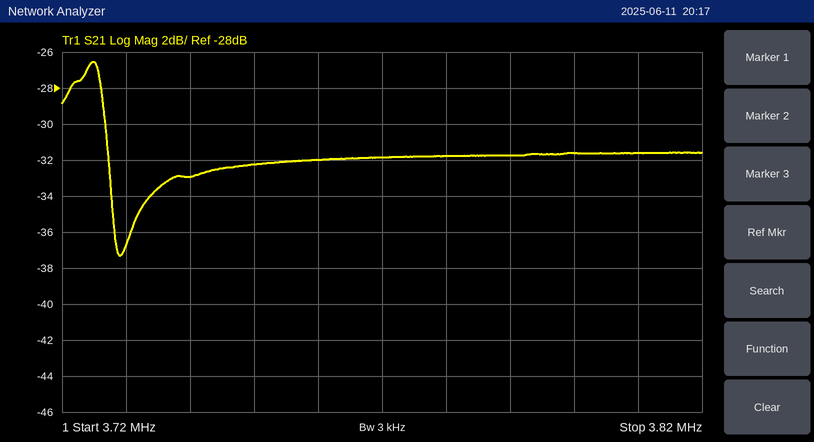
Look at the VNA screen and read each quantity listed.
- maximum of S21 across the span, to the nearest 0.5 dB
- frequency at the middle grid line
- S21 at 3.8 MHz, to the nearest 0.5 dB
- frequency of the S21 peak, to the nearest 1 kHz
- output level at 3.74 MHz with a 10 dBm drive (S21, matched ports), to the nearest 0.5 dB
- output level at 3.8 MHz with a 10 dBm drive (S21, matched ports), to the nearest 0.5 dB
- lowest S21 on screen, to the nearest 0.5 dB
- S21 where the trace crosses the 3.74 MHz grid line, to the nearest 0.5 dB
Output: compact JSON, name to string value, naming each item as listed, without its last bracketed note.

{"maximum of S21 across the span, to the nearest 0.5 dB": "-26.5 dB", "frequency at the middle grid line": "3.77 MHz", "S21 at 3.8 MHz, to the nearest 0.5 dB": "-31.5 dB", "frequency of the S21 peak, to the nearest 1 kHz": "3.725 MHz", "output level at 3.74 MHz with a 10 dBm drive (S21, matched ports), to the nearest 0.5 dB": "-23.0 dBm", "output level at 3.8 MHz with a 10 dBm drive (S21, matched ports), to the nearest 0.5 dB": "-21.5 dBm", "lowest S21 on screen, to the nearest 0.5 dB": "-37.5 dB", "S21 where the trace crosses the 3.74 MHz grid line, to the nearest 0.5 dB": "-33.0 dB"}
